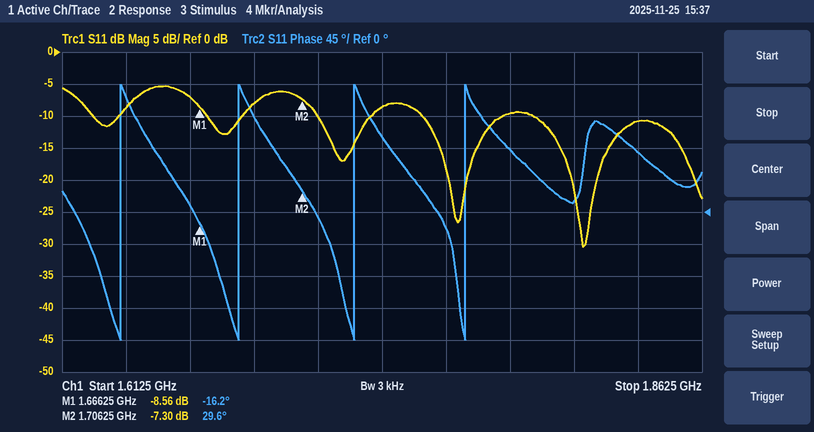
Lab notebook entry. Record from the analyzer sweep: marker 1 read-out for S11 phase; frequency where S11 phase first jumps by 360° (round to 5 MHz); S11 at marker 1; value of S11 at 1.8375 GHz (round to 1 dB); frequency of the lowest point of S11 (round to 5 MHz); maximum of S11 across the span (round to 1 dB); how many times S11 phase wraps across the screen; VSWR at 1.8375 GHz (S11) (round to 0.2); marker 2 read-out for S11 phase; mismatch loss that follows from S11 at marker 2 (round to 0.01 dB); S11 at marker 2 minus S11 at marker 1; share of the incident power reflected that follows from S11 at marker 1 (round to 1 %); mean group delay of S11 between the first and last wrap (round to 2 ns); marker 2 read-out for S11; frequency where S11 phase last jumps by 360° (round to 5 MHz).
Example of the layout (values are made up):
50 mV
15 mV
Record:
-16.2°
1.635 GHz
-8.56 dB
-11 dB
1.815 GHz
-5 dB
4
1.8
29.6°
0.89 dB
1.26 dB
14 %
22 ns
-7.30 dB
1.770 GHz
